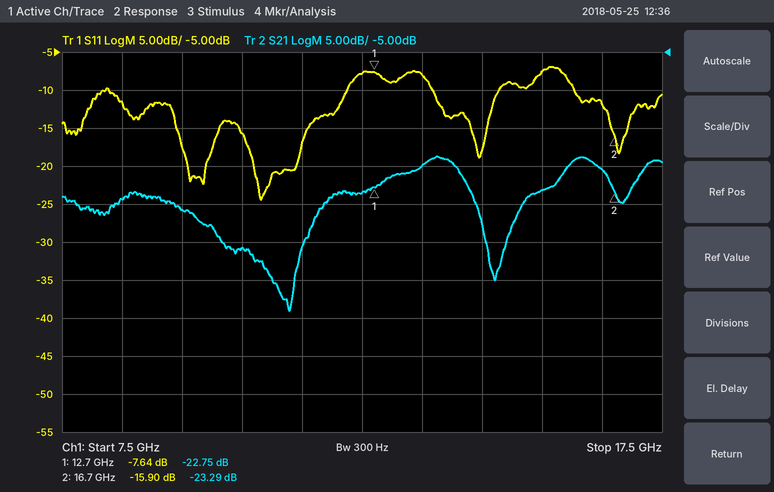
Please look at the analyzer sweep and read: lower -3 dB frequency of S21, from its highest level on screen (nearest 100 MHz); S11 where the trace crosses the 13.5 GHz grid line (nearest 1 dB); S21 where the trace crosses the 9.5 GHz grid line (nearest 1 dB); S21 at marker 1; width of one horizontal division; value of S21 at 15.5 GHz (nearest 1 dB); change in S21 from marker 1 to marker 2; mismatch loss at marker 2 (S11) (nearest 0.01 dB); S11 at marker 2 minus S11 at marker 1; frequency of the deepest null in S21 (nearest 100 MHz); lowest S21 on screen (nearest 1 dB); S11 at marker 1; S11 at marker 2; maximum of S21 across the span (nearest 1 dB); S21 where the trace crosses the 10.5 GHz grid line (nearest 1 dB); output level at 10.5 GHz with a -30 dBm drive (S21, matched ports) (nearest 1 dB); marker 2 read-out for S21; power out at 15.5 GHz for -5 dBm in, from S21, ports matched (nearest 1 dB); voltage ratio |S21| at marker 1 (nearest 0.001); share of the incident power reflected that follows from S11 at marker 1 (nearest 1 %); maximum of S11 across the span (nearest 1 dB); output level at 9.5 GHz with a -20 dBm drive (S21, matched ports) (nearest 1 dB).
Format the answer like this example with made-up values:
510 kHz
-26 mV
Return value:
12.9 GHz
-8 dB
-26 dB
-22.75 dB
1 GHz
-23 dB
-0.54 dB
0.11 dB
-8.26 dB
11.3 GHz
-39 dB
-7.64 dB
-15.90 dB
-19 dB
-31 dB
-61 dBm
-23.29 dB
-28 dBm
0.073
17 %
-7 dB
-46 dBm
